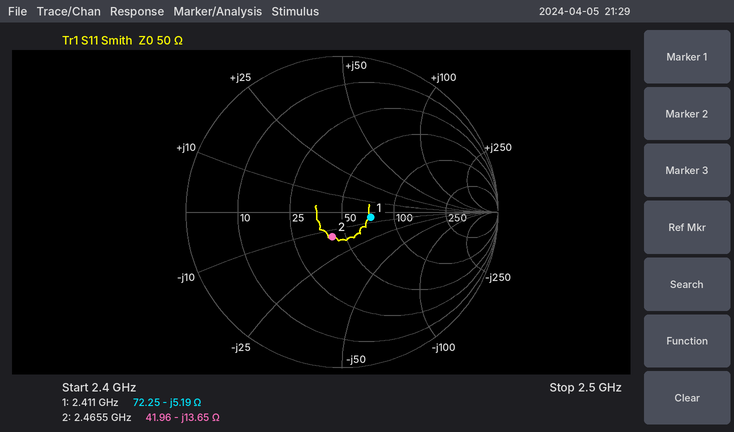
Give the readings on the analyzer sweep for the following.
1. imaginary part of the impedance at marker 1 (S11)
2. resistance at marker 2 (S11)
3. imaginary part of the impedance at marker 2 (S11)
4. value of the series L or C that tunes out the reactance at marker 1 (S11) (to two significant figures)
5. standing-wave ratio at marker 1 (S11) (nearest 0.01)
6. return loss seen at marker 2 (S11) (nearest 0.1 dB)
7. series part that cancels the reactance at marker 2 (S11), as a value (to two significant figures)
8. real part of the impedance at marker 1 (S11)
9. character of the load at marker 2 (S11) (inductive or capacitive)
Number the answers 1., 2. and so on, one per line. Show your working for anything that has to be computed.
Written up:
1. -5.19 Ω
2. 41.96 Ω
3. -13.65 Ω
4. L = 5.19 Ω/(2π × 2.411 GHz) ≈ 343 pH, so 340 pH to two significant figures
5. 1.46
6. 15.4 dB
7. L = 13.65 Ω/(2π × 2.4655 GHz) ≈ 881 pH, so 880 pH to two significant figures
8. 72.25 Ω
9. capacitive
